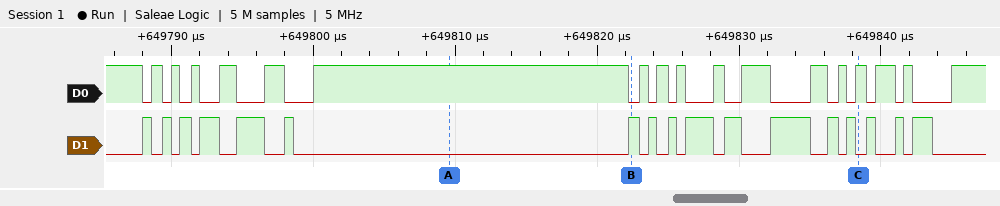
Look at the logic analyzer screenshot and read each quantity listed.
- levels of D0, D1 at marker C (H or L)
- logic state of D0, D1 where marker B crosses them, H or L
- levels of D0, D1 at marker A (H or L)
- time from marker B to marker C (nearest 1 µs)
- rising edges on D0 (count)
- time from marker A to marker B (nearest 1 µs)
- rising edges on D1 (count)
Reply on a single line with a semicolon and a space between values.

D0=H, D1=L; D0=L, D1=H; D0=H, D1=L; 16 µs; 17; 13 µs; 17
